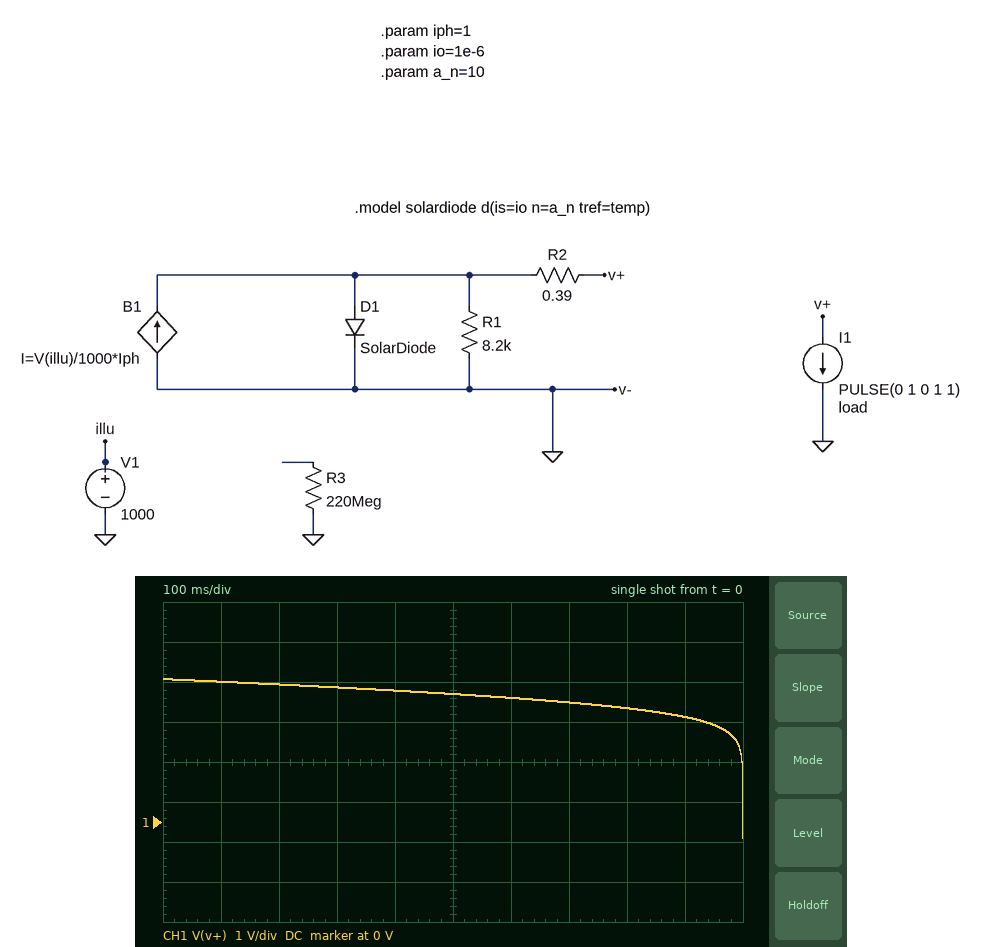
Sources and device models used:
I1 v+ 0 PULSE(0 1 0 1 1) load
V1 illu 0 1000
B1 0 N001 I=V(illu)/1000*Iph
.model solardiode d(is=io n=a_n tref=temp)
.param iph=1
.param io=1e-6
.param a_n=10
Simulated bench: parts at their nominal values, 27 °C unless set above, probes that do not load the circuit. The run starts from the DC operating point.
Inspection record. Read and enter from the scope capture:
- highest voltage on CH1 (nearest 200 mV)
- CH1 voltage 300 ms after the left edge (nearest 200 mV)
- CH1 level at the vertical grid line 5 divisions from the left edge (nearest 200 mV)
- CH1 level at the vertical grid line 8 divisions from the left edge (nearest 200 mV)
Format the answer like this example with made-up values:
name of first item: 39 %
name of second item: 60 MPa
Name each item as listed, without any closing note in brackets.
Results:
highest voltage on CH1: 3.6 V
CH1 voltage 300 ms after the left edge: 3.4 V
CH1 level at the vertical grid line 5 divisions from the left edge: 3.2 V
CH1 level at the vertical grid line 8 divisions from the left edge: 2.8 V
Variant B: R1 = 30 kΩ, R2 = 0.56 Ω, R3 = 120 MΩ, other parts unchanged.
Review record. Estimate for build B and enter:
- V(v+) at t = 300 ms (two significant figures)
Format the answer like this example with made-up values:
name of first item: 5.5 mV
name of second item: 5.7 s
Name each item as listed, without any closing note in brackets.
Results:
V(v+) at t = 300 ms: 3.3 V
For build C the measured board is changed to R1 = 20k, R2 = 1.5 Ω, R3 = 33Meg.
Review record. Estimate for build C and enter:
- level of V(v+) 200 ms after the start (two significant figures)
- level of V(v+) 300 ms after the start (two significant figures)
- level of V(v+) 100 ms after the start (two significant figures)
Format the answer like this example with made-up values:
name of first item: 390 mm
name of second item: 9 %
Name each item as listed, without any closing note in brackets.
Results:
level of V(v+) 200 ms after the start: 3.2 V
level of V(v+) 300 ms after the start: 3.0 V
level of V(v+) 100 ms after the start: 3.4 V
